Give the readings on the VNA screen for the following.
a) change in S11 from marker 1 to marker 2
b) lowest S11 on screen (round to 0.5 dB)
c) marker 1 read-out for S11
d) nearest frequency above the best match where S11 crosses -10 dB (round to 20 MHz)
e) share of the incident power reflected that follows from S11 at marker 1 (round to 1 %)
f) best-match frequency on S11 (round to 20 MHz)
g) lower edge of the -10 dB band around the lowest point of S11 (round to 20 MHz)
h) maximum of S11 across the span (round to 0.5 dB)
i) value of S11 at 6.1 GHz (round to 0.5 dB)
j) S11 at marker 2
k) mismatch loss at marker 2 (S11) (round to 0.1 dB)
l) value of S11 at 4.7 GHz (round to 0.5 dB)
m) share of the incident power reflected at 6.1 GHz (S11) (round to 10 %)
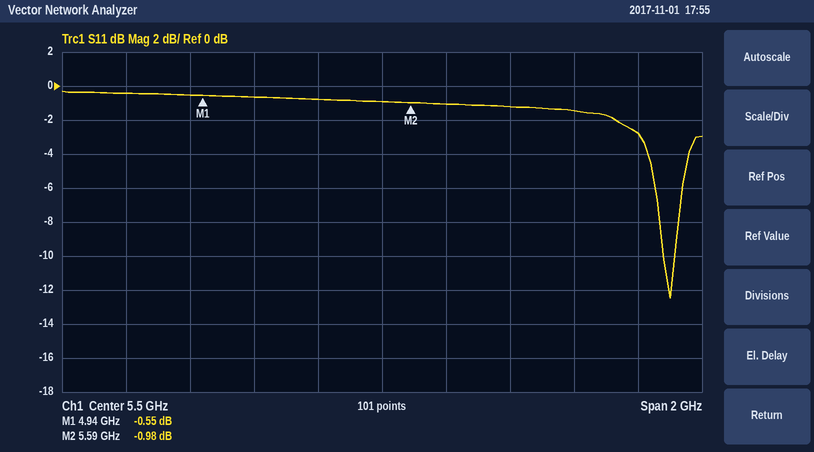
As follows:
-0.43 dB
-12.5 dB
-0.55 dB
6.42 GHz
88 %
6.40 GHz
6.38 GHz
-0.5 dB
-1.5 dB
-0.98 dB
6.9 dB
-0.5 dB
70 %
